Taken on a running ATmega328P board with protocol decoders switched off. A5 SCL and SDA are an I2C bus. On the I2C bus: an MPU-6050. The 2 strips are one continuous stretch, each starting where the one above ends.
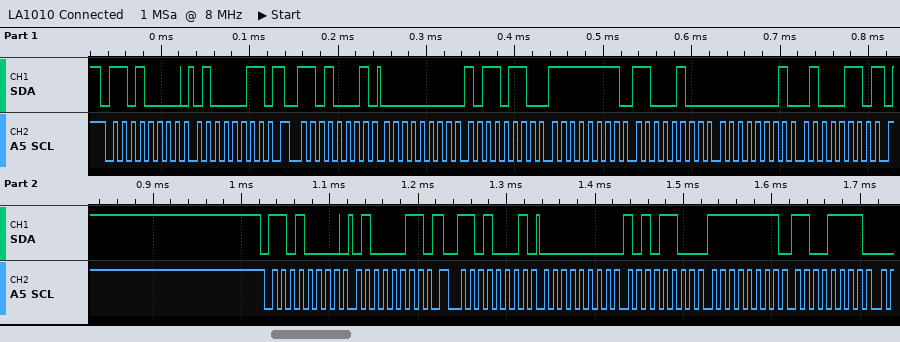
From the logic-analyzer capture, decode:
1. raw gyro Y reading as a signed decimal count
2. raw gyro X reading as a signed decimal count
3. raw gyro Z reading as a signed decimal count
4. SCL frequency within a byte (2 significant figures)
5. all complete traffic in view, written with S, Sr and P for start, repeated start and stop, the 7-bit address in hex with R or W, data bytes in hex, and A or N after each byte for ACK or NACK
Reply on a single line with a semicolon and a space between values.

-60; 182; 326; 100 kHz; S 68W A 43 A Sr 68R A 00 A B6 A FF A C4 A 01 A 46 N P S 68W A 43 A Sr 68R A 00 A AC A FF A CF A
